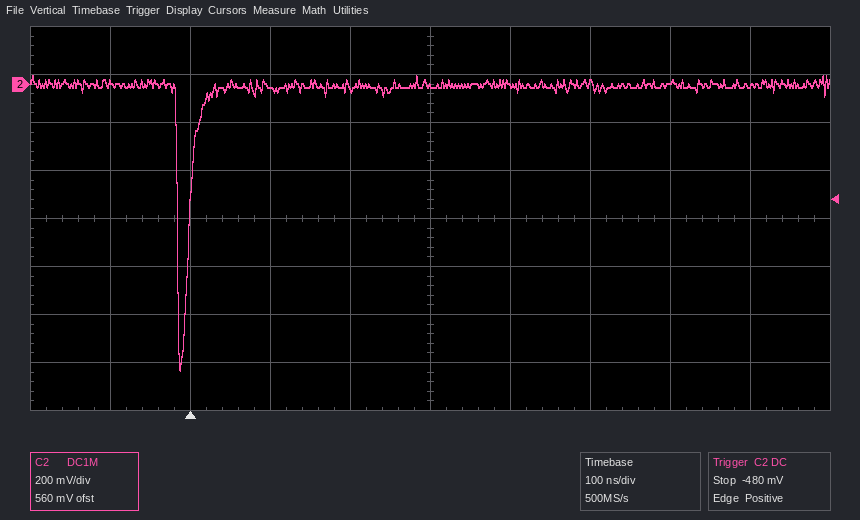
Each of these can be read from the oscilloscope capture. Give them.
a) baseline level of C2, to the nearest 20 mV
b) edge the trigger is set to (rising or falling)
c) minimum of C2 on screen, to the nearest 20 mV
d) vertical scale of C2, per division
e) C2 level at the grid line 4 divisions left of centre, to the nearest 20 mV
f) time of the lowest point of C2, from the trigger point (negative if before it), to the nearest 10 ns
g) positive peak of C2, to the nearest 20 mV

0 mV
rising
-1.20 V
200 mV
0 mV
-10 ns
40 mV
